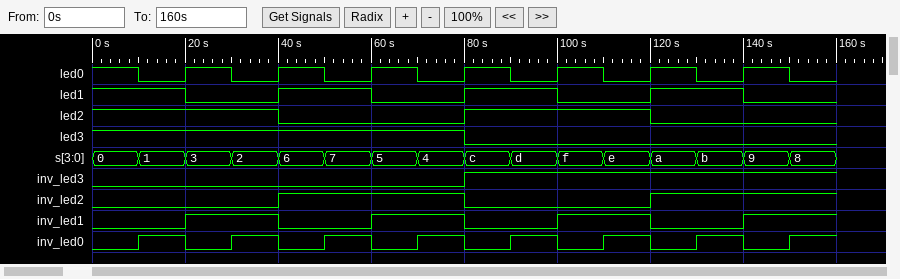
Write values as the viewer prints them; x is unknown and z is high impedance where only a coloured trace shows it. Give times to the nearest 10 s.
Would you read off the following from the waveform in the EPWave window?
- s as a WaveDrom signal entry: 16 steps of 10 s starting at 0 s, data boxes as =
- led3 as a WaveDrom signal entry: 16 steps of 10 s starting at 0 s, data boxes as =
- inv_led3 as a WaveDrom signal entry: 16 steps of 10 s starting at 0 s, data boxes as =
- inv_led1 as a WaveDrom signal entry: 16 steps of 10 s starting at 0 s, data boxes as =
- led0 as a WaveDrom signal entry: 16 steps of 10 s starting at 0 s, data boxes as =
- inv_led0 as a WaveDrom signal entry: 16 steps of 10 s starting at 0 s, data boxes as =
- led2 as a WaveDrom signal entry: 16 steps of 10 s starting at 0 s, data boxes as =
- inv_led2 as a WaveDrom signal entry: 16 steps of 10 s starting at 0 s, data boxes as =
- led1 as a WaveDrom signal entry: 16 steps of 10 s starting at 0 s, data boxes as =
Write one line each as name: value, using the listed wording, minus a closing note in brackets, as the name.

s as a WaveDrom signal entry: 16 steps of 10 s starting at 0 s, data boxes as =: {name: 's', wave: '================', data: '0 1 3 2 6 7 5 4 c d f e a b 9 8'}
led3 as a WaveDrom signal entry: 16 steps of 10 s starting at 0 s, data boxes as =: {name: 'led3', wave: '1.......0.......'}
inv_led3 as a WaveDrom signal entry: 16 steps of 10 s starting at 0 s, data boxes as =: {name: 'inv_led3', wave: '0.......1.......'}
inv_led1 as a WaveDrom signal entry: 16 steps of 10 s starting at 0 s, data boxes as =: {name: 'inv_led1', wave: '0.1.0.1.0.1.0.1.'}
led0 as a WaveDrom signal entry: 16 steps of 10 s starting at 0 s, data boxes as =: {name: 'led0', wave: '1010101010101010'}
inv_led0 as a WaveDrom signal entry: 16 steps of 10 s starting at 0 s, data boxes as =: {name: 'inv_led0', wave: '0101010101010101'}
led2 as a WaveDrom signal entry: 16 steps of 10 s starting at 0 s, data boxes as =: {name: 'led2', wave: '1...0...1...0...'}
inv_led2 as a WaveDrom signal entry: 16 steps of 10 s starting at 0 s, data boxes as =: {name: 'inv_led2', wave: '0...1...0...1...'}
led1 as a WaveDrom signal entry: 16 steps of 10 s starting at 0 s, data boxes as =: {name: 'led1', wave: '1.0.1.0.1.0.1.0.'}
